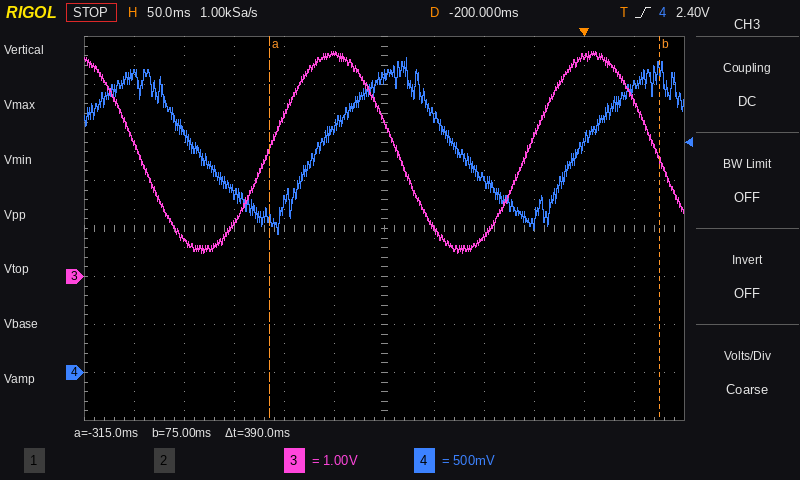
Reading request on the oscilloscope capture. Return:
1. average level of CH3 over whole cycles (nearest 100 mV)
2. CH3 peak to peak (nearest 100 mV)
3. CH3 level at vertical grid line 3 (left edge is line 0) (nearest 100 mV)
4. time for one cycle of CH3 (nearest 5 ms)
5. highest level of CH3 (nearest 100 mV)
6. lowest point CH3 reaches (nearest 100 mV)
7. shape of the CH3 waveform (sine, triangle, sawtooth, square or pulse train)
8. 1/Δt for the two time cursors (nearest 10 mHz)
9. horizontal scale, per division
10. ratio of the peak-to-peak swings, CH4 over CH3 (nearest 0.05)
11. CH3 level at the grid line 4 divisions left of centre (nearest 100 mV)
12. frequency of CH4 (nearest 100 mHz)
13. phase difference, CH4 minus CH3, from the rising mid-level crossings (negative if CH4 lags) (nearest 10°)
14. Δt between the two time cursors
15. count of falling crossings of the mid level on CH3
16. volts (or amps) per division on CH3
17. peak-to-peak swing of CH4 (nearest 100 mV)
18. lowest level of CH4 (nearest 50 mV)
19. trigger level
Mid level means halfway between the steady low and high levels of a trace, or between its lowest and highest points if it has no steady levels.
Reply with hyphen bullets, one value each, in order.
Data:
- 2.6 V
- 4.2 V
- 1.1 V
- 260 ms
- 4.7 V
- 500 mV
- sine
- 2.56 Hz
- 50 ms
- 0.45
- 800 mV
- 3.8 Hz
- -70°
- 390 ms
- 3
- 1 V
- 1.80 V
- 1.45 V
- 2.40 V
